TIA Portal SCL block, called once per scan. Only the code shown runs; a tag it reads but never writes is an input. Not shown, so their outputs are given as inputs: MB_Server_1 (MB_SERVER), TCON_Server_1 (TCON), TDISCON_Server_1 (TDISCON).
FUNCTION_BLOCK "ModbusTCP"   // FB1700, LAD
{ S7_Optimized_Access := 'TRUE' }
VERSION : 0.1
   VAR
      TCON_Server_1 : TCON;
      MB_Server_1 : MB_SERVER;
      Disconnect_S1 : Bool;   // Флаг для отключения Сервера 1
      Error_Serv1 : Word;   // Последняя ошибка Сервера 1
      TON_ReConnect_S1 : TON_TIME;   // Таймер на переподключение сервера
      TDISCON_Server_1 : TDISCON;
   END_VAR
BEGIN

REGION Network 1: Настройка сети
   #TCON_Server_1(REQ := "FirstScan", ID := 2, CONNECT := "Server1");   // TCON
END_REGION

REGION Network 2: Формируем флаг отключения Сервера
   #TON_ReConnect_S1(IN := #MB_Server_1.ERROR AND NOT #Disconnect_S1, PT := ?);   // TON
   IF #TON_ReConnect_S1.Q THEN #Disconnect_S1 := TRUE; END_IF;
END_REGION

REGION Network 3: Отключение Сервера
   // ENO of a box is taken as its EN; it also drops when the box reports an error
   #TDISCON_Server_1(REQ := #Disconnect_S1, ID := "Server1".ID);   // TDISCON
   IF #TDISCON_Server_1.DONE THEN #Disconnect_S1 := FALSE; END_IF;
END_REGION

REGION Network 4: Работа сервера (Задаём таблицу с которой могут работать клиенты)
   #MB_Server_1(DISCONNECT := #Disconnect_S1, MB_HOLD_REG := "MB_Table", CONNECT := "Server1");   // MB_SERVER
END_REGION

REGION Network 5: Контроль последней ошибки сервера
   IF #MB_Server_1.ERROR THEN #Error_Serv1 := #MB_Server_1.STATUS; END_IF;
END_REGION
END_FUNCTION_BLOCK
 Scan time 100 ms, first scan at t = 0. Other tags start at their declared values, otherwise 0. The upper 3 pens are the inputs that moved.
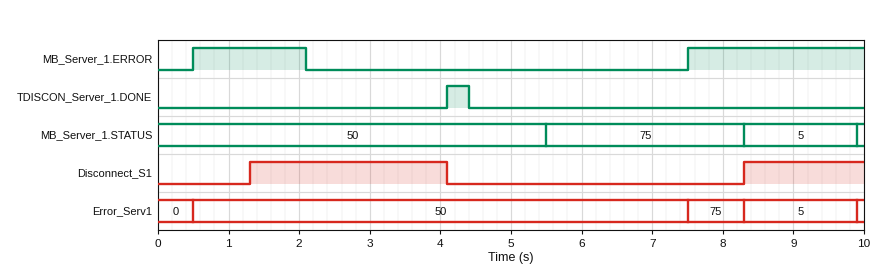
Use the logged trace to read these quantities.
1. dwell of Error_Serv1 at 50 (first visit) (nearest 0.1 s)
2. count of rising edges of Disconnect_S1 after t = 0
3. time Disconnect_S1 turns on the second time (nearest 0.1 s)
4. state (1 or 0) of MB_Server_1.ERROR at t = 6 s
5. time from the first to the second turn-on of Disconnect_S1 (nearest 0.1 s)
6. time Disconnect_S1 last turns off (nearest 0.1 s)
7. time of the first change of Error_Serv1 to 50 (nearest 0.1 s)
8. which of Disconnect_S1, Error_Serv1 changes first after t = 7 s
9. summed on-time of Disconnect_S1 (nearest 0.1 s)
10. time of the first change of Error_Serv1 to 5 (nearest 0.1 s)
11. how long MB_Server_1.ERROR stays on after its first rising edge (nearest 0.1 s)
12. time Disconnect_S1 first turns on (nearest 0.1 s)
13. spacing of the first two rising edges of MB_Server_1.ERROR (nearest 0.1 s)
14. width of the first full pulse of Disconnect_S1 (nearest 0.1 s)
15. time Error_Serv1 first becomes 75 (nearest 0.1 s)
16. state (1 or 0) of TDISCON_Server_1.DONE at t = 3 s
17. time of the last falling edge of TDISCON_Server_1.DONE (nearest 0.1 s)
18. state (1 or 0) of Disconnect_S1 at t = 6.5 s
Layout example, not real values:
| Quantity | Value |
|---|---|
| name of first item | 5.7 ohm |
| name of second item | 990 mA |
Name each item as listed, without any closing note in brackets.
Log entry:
| Quantity | Value |
|---|---|
| dwell of Error_Serv1 at 50 (first visit) | 7.0 s |
| count of rising edges of Disconnect_S1 after t = 0 | 2 |
| time Disconnect_S1 turns on the second time | 8.3 s |
| state (1 or 0) of MB_Server_1.ERROR at t = 6 s | 0 |
| time from the first to the second turn-on of Disconnect_S1 | 7.0 s |
| time Disconnect_S1 last turns off | 4.1 s |
| time of the first change of Error_Serv1 to 50 | 0.5 s |
| which of Disconnect_S1, Error_Serv1 changes first after t = 7 s | Error_Serv1 |
| summed on-time of Disconnect_S1 | 4.5 s |
| time of the first change of Error_Serv1 to 5 | 8.3 s |
| how long MB_Server_1.ERROR stays on after its first rising edge | 1.6 s |
| time Disconnect_S1 first turns on | 1.3 s |
| spacing of the first two rising edges of MB_Server_1.ERROR | 7.0 s |
| width of the first full pulse of Disconnect_S1 | 2.8 s |
| time Error_Serv1 first becomes 75 | 7.5 s |
| state (1 or 0) of TDISCON_Server_1.DONE at t = 3 s | 0 |
| time of the last falling edge of TDISCON_Server_1.DONE | 4.4 s |
| state (1 or 0) of Disconnect_S1 at t = 6.5 s | 0 |
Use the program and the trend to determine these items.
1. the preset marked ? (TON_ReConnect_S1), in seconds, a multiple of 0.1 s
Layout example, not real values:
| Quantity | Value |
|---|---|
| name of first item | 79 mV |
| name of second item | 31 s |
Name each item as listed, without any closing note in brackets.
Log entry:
| Quantity | Value |
|---|---|
| the preset marked ? (TON_ReConnect_S1), in seconds, a multiple of 0.1 s | 0.8 s |
